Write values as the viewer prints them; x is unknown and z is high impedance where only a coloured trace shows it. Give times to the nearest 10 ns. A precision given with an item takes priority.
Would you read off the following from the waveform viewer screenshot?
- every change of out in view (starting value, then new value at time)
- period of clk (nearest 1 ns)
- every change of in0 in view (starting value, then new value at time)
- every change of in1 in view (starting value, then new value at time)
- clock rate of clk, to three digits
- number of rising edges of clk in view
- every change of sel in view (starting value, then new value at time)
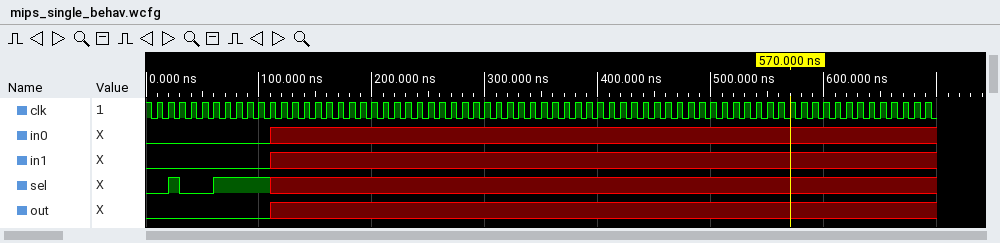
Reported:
0, x at 110 ns
10 ns
0, x at 110 ns
0, x at 110 ns
100 MHz
69
0, 1 at 20 ns, 0 at 30 ns, 1 at 60 ns, x at 110 ns
